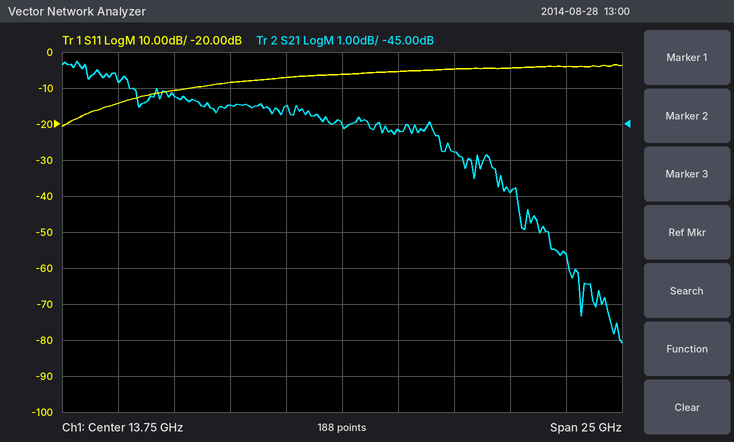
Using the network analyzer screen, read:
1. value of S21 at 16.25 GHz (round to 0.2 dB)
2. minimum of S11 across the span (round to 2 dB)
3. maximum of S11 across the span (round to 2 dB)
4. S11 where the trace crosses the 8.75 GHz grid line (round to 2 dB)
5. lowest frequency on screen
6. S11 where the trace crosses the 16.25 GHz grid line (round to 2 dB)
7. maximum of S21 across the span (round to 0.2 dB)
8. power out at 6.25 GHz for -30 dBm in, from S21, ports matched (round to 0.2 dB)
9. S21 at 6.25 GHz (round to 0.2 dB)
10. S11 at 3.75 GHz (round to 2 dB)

-45.2 dB
-20 dB
-4 dB
-8 dB
1.25 GHz
-6 dB
-43.2 dB
-74.2 dBm
-44.2 dB
-14 dB
